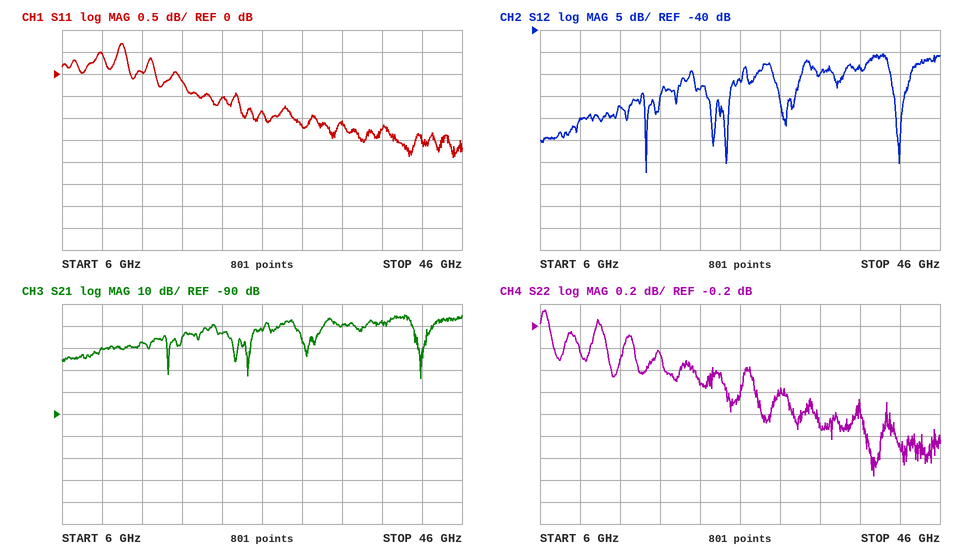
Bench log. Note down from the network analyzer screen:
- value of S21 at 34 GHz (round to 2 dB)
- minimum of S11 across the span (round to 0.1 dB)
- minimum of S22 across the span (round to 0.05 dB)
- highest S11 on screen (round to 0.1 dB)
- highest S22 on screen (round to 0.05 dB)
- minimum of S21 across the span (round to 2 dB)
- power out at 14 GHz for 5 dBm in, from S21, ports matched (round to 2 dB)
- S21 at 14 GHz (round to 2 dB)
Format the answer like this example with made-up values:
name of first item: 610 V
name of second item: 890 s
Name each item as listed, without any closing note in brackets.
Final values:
value of S21 at 34 GHz: -50 dB
minimum of S11 across the span: -1.9 dB
minimum of S22 across the span: -1.55 dB
highest S11 on screen: 0.7 dB
highest S22 on screen: -0.05 dB
minimum of S21 across the span: -74 dB
power out at 14 GHz for 5 dBm in, from S21, ports matched: -52 dBm
S21 at 14 GHz: -58 dB
